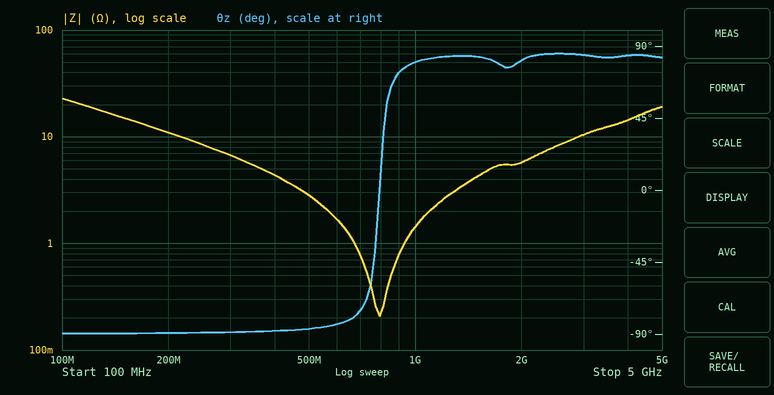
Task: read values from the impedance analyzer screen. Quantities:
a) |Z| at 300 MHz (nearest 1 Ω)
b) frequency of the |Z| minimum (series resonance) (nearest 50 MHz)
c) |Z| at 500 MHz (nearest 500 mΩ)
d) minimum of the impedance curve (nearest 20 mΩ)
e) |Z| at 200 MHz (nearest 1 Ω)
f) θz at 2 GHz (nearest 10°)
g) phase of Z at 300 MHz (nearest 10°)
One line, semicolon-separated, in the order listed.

7 Ω; 800 MHz; 3.0 Ω; 200 mΩ; 11 Ω; 80°; -90°
